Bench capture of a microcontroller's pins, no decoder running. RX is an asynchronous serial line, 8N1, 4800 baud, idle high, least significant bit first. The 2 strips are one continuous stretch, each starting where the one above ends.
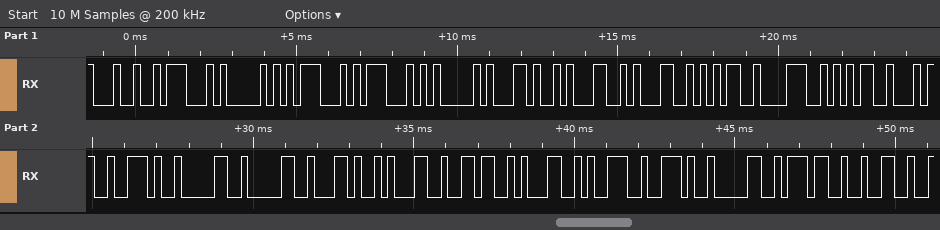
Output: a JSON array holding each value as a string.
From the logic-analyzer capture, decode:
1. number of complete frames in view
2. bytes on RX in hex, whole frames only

["25", "24 47 50 47 47 41 2C 31 31 35 38 35 34 2E 30 30 2C 31 36 31 39 2E 30 37 32"]
